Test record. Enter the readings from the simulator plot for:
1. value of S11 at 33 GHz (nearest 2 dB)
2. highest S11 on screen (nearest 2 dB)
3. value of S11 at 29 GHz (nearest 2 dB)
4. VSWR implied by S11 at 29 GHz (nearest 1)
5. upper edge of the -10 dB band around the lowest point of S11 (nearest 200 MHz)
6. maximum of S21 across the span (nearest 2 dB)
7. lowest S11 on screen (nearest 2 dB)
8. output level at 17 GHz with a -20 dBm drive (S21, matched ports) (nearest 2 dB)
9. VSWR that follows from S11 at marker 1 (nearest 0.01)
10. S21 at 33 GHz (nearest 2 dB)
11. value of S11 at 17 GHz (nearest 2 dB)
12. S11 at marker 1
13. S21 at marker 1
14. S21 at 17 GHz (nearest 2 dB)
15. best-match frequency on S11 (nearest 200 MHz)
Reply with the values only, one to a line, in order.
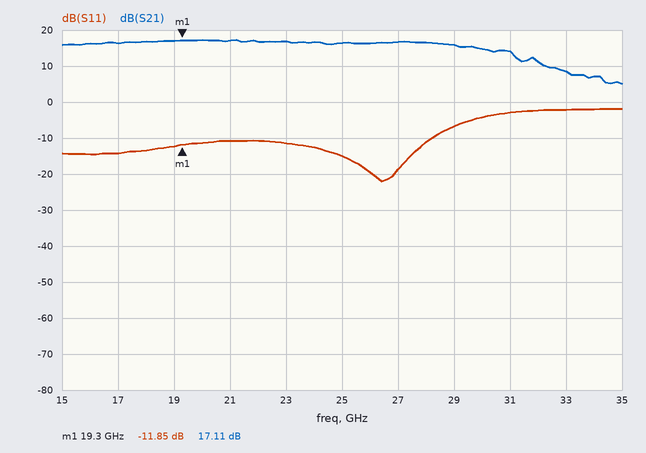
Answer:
-2 dB
-2 dB
-6 dB
3
28.2 GHz
18 dB
-22 dB
-4 dBm
1.69
8 dB
-14 dB
-11.85 dB
17.11 dB
16 dB
26.4 GHz
